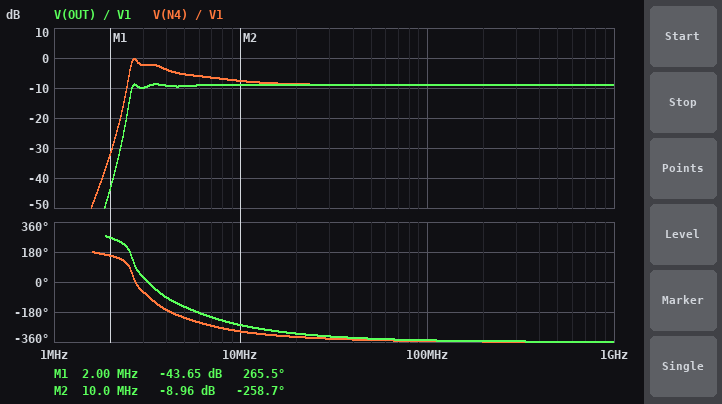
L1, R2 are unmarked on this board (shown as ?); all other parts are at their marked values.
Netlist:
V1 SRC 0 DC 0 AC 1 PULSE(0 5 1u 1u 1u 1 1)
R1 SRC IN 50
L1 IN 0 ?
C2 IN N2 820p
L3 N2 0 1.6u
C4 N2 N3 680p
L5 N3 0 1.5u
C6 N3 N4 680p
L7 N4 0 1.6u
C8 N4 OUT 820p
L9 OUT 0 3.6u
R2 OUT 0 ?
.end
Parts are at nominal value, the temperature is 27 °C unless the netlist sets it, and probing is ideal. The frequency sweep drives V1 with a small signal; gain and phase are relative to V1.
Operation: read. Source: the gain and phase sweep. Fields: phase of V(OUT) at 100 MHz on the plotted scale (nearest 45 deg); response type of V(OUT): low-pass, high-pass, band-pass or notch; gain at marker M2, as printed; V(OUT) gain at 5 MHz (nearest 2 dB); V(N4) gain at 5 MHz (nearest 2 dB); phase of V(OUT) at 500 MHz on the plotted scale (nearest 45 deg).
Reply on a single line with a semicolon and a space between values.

-360 deg; high-pass; -8.96 dB; -10 dB; -6 dB; -360 deg
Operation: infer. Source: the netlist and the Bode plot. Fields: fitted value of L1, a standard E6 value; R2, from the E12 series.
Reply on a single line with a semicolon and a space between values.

10 µH; 27 Ω
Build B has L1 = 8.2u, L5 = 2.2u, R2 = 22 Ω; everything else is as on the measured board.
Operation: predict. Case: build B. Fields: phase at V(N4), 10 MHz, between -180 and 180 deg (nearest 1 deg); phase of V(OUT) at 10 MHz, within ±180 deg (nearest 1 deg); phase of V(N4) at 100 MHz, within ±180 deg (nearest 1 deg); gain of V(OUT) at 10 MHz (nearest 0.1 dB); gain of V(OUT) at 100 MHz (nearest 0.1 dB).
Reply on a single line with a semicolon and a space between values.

52 deg; 96 deg; 5 deg; -10.4 dB; -10.3 dB
